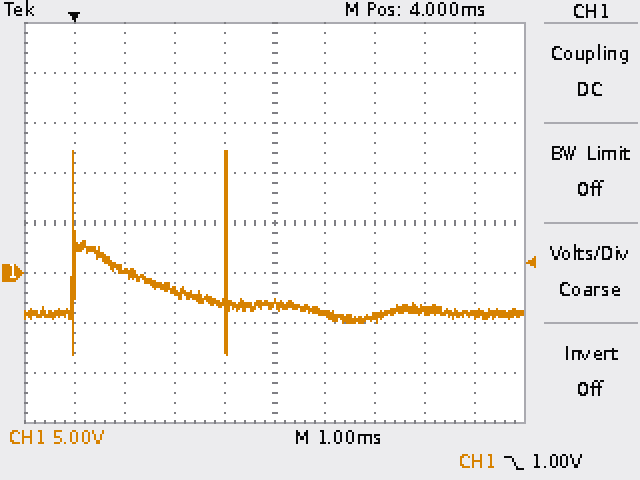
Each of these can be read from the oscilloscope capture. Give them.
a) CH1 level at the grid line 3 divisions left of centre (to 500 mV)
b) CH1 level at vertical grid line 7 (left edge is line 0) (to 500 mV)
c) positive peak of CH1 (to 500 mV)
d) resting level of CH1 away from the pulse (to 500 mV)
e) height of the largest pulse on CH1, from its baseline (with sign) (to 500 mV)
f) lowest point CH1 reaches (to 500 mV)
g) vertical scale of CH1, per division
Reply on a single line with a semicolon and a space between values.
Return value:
500 mV; -4.5 V; 12.0 V; -4.0 V; +16.0 V; -8.0 V; 5 V
